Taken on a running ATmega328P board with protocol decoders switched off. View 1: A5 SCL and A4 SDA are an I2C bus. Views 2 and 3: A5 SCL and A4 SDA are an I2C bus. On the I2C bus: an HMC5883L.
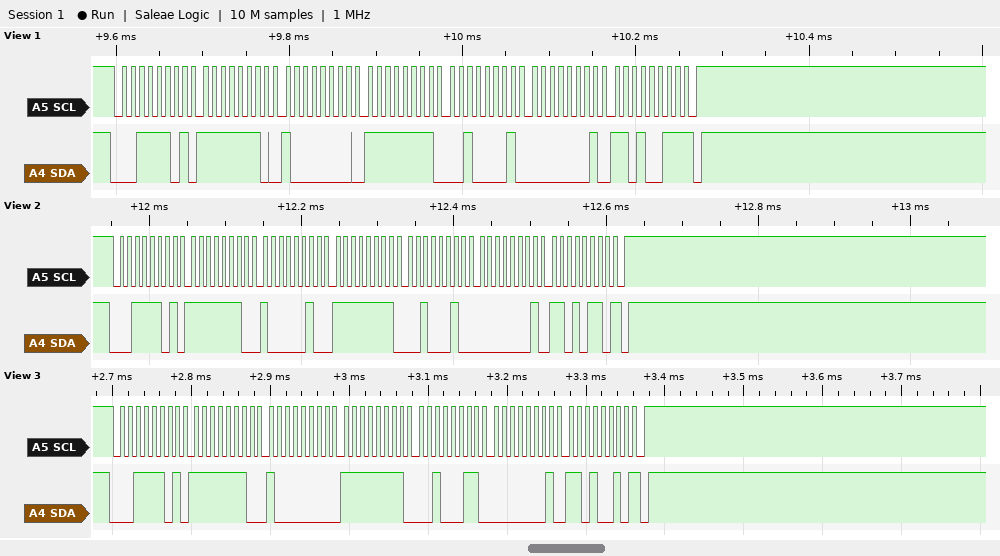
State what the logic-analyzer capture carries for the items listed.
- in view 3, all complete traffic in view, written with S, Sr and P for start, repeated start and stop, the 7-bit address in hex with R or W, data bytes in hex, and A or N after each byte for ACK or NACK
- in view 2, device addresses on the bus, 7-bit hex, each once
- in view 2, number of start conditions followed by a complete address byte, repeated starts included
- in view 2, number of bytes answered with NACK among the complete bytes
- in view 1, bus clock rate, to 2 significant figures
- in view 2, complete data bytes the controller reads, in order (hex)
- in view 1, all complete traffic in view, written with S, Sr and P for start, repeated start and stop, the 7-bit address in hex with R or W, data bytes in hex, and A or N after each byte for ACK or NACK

S 1ER A FE A 80 A FF A 23 A 01 A D2 N P
0x1E
1
1
100 kHz
FE 82 FF 22 01 D6
S 1ER A FE A 80 A FF A 21 A 01 A D3 N P
